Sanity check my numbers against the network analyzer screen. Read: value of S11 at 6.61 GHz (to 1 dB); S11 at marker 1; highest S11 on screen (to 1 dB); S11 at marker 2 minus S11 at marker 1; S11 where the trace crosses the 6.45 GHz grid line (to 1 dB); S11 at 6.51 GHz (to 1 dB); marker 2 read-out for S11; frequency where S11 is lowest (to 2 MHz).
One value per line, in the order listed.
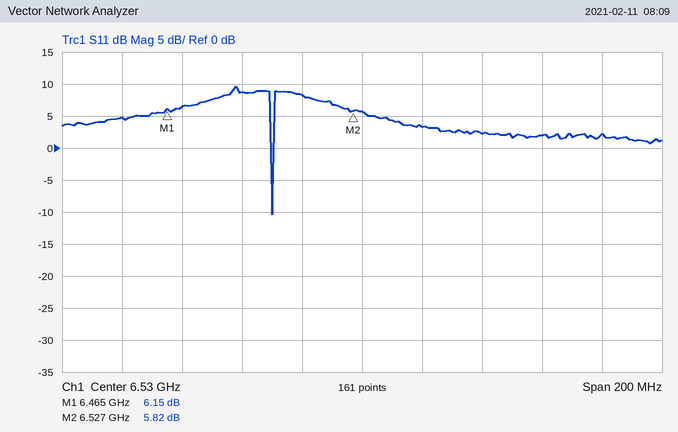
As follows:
2 dB
6.15 dB
10 dB
-0.33 dB
5 dB
8 dB
5.82 dB
6.500 GHz
